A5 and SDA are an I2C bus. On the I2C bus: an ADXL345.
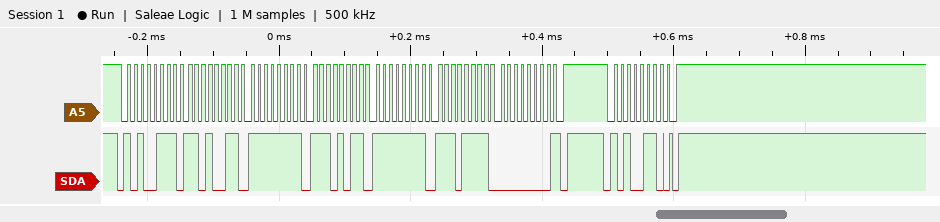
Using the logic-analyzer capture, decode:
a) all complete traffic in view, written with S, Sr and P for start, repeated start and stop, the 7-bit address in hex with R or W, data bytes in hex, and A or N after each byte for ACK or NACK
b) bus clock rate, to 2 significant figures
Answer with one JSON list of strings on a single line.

["S 53R A D3 A FF A EB A FF A EF A 00 N P S 53W A P", "100 kHz"]
